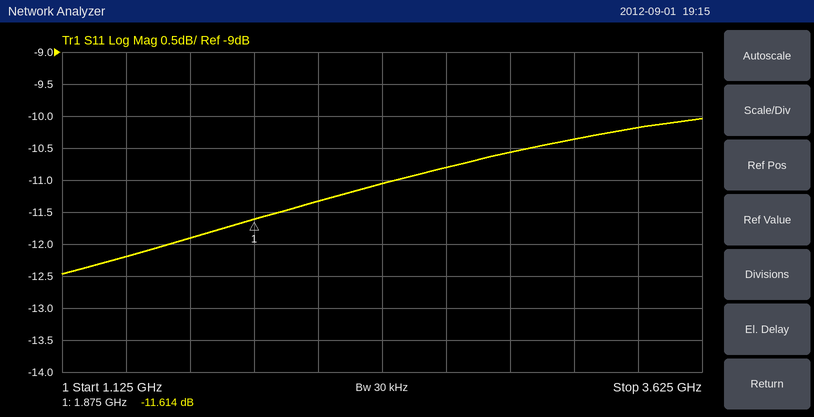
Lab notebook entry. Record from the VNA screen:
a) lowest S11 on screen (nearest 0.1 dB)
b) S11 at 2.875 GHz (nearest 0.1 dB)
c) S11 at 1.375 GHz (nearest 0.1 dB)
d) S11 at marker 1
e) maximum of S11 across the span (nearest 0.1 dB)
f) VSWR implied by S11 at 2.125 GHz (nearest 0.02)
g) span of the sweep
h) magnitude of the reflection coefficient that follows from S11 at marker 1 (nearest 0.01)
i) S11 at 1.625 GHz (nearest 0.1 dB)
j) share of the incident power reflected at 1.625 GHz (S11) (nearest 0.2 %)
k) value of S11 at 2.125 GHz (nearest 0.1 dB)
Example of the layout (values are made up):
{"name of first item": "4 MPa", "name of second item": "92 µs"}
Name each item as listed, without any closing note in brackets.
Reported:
{"lowest S11 on screen": "-12.5 dB", "S11 at 2.875 GHz": "-10.6 dB", "S11 at 1.375 GHz": "-12.2 dB", "S11 at marker 1": "-11.614 dB", "maximum of S11 across the span": "-10.0 dB", "VSWR implied by S11 at 2.125 GHz": "1.74", "span of the sweep": "2.5 GHz", "magnitude of the reflection coefficient that follows from S11 at marker 1": "0.26", "S11 at 1.625 GHz": "-11.9 dB", "share of the incident power reflected at 1.625 GHz (S11)": "6.4 %", "value of S11 at 2.125 GHz": "-11.3 dB"}
